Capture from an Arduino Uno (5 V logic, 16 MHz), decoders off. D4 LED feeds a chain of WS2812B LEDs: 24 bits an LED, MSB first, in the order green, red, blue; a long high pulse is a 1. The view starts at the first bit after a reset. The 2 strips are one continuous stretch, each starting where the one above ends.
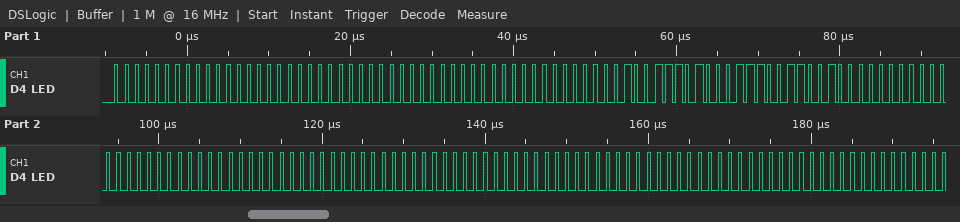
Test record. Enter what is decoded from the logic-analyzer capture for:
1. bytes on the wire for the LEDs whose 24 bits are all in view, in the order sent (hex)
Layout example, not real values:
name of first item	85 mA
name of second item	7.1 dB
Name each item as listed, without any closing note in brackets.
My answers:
bytes on the wire for the LEDs whose 24 bits are all in view, in the order sent	00 00 00 00 00 00 27 47 32 00 00 00 00 00 00 00 00 00
